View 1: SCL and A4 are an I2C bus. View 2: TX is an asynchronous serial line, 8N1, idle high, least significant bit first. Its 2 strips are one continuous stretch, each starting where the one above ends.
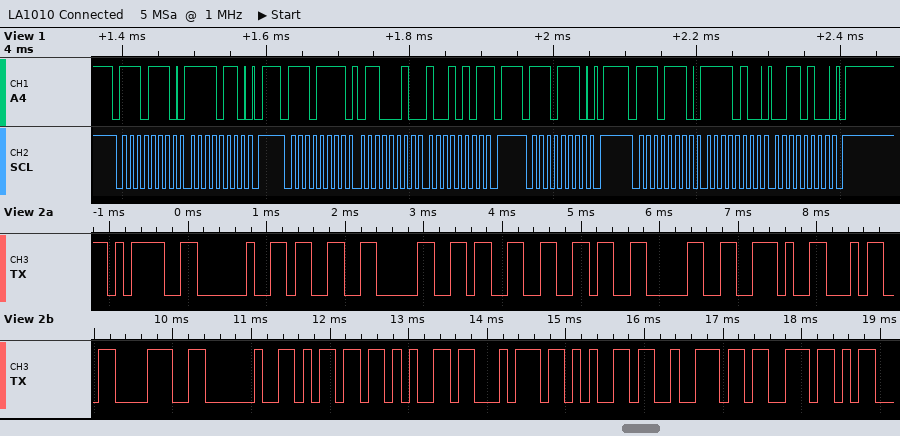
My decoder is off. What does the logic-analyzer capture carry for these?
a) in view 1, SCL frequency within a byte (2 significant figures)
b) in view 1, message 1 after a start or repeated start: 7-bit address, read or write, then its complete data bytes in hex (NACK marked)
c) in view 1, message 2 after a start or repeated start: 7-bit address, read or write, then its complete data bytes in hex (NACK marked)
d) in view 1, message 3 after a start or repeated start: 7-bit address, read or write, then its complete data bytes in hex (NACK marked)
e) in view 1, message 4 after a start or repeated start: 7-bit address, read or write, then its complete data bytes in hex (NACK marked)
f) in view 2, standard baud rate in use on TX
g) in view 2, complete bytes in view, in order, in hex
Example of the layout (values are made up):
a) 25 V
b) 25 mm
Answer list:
a) 100 kHz
b) 0x77 write: F6
c) 0x77 read: 62 95 NACK
d) 0x77 write
e) 0x77 write: F4 34
f) 9600 baud
g) 0x3D 0x20 0x33 0x30 0x33 0x36 0x30 0x2E 0x34 0x38 0x20 0x6D 0x65 0x74 0x65 0x72 0x73
